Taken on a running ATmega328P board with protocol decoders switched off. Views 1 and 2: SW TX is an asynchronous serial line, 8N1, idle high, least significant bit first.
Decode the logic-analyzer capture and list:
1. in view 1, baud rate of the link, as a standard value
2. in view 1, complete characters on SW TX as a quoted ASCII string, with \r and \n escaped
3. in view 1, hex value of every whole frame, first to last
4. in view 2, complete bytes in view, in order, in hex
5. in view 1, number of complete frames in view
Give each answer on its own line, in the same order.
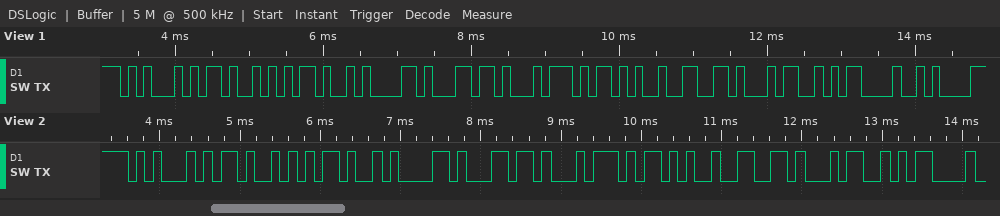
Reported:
9600 baud
"EK-alt+f4\r\n"
45 4B 2D 61 6C 74 2B 66 34 0D 0A
45 4B 2D 61 6C 74 2B 66 34 0D
11
